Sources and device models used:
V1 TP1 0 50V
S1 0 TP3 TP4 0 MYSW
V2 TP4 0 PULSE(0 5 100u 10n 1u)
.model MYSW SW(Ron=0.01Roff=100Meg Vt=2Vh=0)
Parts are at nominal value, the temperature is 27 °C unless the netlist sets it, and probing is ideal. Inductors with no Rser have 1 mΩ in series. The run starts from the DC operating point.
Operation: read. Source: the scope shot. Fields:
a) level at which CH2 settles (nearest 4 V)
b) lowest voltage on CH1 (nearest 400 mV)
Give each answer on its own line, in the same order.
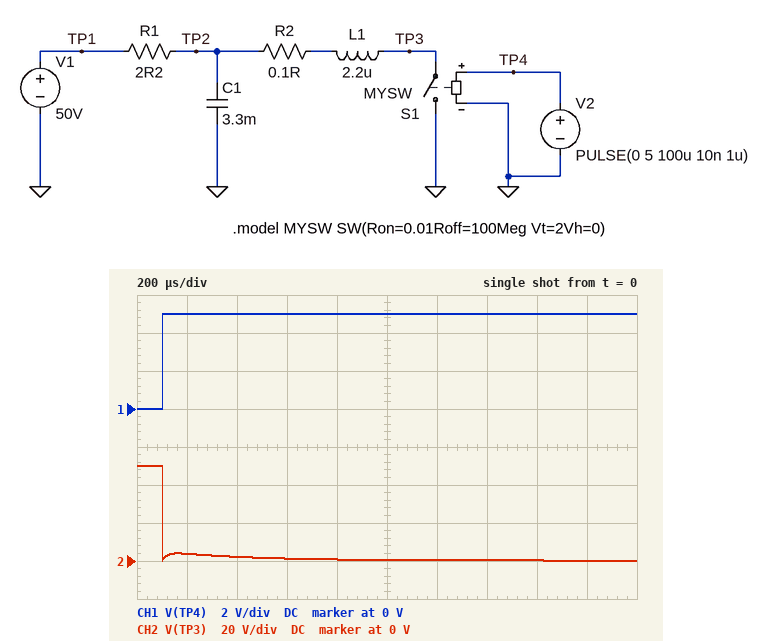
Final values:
0 V
0 V
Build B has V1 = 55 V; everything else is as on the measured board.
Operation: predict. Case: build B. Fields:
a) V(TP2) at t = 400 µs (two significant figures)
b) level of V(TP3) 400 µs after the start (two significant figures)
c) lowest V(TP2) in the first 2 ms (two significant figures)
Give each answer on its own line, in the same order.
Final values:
25 V
2.4 V
2.8 V
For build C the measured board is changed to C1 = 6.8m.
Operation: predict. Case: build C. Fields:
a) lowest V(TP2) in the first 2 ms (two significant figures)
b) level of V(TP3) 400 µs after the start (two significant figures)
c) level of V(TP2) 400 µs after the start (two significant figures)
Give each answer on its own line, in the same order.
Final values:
5.6 V
3.2 V
34 V
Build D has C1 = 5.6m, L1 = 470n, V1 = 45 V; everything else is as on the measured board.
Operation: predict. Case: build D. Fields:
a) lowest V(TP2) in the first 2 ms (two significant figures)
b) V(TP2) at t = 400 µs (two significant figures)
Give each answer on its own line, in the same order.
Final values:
3.9 V
28 V
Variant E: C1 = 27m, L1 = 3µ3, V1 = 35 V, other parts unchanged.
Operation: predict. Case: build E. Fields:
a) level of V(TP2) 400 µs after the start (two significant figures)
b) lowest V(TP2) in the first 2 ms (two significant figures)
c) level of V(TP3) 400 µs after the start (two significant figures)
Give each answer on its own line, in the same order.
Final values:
32 V
19 V
2.9 V
